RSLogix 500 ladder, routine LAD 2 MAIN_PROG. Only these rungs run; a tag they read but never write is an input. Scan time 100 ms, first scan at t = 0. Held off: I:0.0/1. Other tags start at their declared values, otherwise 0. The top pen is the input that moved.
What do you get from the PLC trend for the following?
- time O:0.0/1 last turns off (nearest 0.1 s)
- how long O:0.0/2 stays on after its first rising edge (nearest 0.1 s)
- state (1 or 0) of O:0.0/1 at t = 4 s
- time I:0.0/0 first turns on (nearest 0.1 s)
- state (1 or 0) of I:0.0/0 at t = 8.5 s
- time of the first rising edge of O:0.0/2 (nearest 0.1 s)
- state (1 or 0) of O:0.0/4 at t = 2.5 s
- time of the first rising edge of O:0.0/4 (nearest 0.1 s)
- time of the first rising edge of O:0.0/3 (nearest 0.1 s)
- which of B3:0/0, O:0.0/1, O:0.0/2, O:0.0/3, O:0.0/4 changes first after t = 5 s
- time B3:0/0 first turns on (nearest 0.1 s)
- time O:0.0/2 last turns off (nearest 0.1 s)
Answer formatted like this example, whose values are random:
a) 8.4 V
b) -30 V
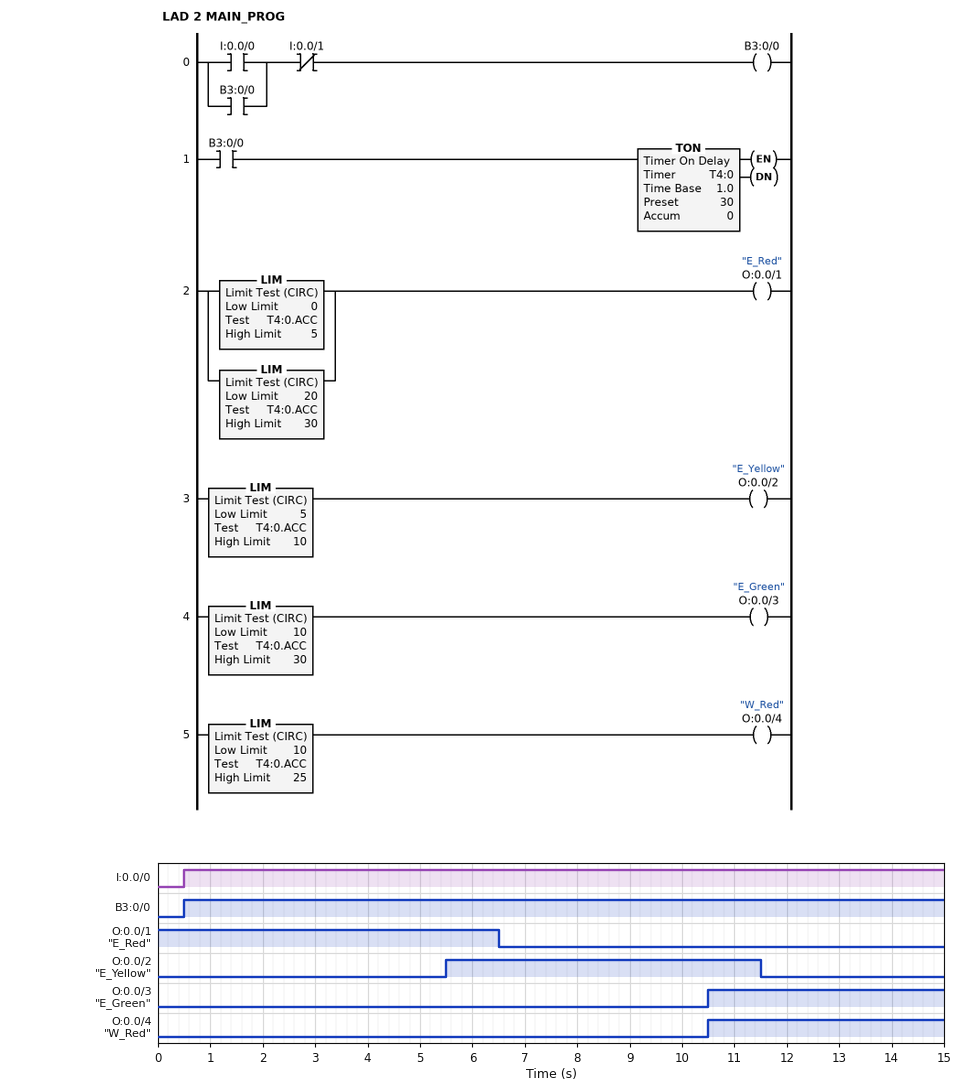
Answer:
a) 6.5 s
b) 6.0 s
c) 1
d) 0.5 s
e) 1
f) 5.5 s
g) 0
h) 10.5 s
i) 10.5 s
j) O:0.0/2
k) 0.5 s
l) 11.5 s
